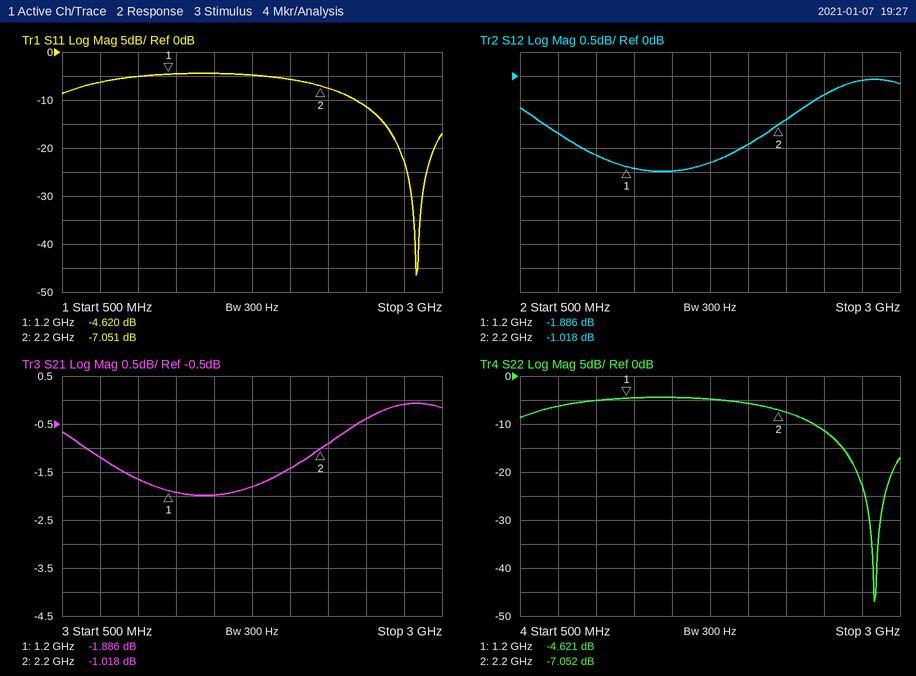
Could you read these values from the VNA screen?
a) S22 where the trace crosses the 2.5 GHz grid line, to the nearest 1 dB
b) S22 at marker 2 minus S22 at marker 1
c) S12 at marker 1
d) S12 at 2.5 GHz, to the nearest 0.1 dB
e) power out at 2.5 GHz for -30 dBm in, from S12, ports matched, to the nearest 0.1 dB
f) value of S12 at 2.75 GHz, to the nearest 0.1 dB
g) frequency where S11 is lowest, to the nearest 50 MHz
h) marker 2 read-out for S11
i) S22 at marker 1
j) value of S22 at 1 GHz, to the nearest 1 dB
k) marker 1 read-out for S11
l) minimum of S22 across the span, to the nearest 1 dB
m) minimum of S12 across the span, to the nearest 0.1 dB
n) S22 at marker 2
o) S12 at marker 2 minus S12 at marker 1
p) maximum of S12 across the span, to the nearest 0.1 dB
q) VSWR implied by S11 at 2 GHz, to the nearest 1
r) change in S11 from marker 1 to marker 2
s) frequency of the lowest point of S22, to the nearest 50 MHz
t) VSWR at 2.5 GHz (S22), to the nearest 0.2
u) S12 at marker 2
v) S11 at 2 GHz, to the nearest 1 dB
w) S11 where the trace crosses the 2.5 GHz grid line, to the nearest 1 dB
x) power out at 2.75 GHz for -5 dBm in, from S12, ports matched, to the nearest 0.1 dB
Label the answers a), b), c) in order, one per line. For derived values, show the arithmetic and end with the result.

a) -11 dB
b) -7.052 − (-4.621) = -2.431 dB
c) -1.886 dB
d) -0.4 dB
e) -30 dBm + (-0.4 dB) = -30.4 dBm
f) -0.1 dB
g) 2.85 GHz
h) -7.051 dB
i) -4.621 dB
j) -5 dB
k) -4.620 dB
l) -47 dB
m) -2.0 dB
n) -7.052 dB
o) -1.018 − (-1.886) = 0.868 dB
p) -0.1 dB
q) |Γ| = 10^(-6/20) = 0.5012; VSWR = (1 + 0.5012)/(1 − 0.5012) ≈ 3
r) -7.051 − (-4.62) = -2.431 dB
s) 2.85 GHz
t) |Γ| = 10^(-11/20) = 0.2818; VSWR = (1 + 0.2818)/(1 − 0.2818) ≈ 1.8
u) -1.018 dB
v) -6 dB
w) -11 dB
x) -5 dBm + (-0.1 dB) = -5.1 dBm
